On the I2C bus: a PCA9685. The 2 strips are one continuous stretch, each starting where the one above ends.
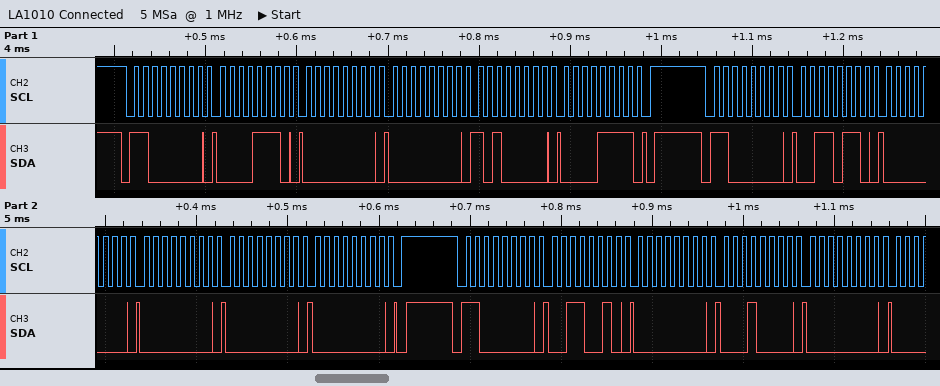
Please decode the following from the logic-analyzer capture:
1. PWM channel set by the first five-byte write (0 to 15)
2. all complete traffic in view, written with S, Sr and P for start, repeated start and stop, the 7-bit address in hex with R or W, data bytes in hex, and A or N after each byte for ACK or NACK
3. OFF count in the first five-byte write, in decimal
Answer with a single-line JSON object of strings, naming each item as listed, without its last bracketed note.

{"PWM channel set by the first five-byte write": "2", "all complete traffic in view, written with S, Sr and P for start, repeated start and stop, the 7-bit address in hex with R or W, data bytes in hex, and A or N after each byte for ACK or NACK": "S 60W A 0E A 00 A 00 A A0 A 0F A P S 60W A 36 A 00 A 00 A 00 A 00 A P S 60W A 32 A 00 A 10 A 00 A", "OFF count in the first five-byte write, in decimal": "4000"}
